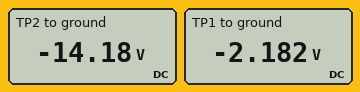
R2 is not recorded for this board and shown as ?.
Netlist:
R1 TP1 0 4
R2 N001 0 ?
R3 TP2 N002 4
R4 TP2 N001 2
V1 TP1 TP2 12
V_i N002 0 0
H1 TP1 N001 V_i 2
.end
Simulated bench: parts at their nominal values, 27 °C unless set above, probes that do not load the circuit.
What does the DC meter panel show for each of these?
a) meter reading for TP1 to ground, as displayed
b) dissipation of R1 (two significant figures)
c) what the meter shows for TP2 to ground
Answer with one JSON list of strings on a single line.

["-2.182 V", "1.2 W", "-14.18 V"]
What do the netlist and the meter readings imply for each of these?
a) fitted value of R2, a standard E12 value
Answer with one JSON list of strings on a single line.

["1.2 Ω"]
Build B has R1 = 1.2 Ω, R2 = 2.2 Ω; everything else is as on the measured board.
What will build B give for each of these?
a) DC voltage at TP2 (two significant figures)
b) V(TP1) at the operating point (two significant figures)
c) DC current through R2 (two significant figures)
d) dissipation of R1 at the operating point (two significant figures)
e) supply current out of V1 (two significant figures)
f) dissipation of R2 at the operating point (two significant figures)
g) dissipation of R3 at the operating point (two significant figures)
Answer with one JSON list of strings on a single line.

["-12 V", "210 mV", "2.8 A", "36 mW", "12 A", "17 W", "35 W"]
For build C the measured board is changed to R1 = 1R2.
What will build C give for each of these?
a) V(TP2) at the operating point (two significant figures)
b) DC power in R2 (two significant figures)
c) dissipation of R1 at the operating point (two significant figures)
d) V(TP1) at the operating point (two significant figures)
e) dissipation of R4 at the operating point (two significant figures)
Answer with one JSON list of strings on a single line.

["-13 V", "24 W", "1.5 W", "-1.3 V", "170 W"]
